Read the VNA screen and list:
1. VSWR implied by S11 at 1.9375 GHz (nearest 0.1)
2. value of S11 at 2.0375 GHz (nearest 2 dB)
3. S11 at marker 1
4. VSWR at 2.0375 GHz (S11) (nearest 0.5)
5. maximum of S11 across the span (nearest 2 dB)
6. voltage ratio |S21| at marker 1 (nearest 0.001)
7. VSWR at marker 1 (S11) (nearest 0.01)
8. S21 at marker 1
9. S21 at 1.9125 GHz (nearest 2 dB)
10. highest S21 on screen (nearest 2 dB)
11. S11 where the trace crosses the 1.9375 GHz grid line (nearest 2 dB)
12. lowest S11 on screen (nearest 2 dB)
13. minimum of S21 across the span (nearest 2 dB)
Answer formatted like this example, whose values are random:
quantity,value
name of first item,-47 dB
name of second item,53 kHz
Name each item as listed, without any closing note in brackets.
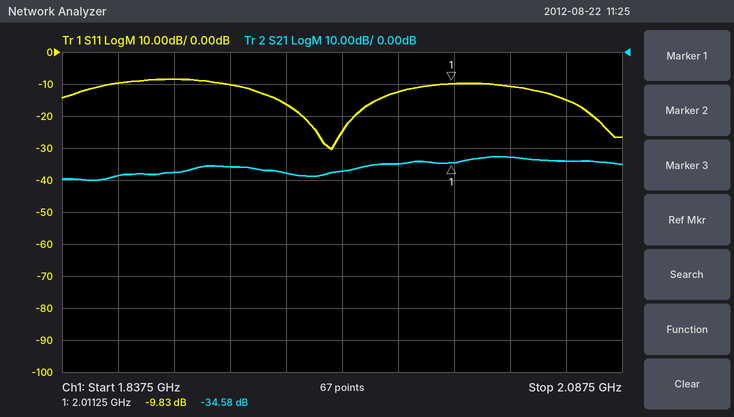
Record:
quantity,value
VSWR implied by S11 at 1.9375 GHz,1.4
value of S11 at 2.0375 GHz,-10 dB
S11 at marker 1,-9.83 dB
VSWR at 2.0375 GHz (S11),2.0
maximum of S11 across the span,-8 dB
voltage ratio |S21| at marker 1,0.019
VSWR at marker 1 (S11),1.95
S21 at marker 1,-34.58 dB
S21 at 1.9125 GHz,-36 dB
highest S21 on screen,-32 dB
S11 where the trace crosses the 1.9375 GHz grid line,-16 dB
lowest S11 on screen,-30 dB
minimum of S21 across the span,-40 dB
